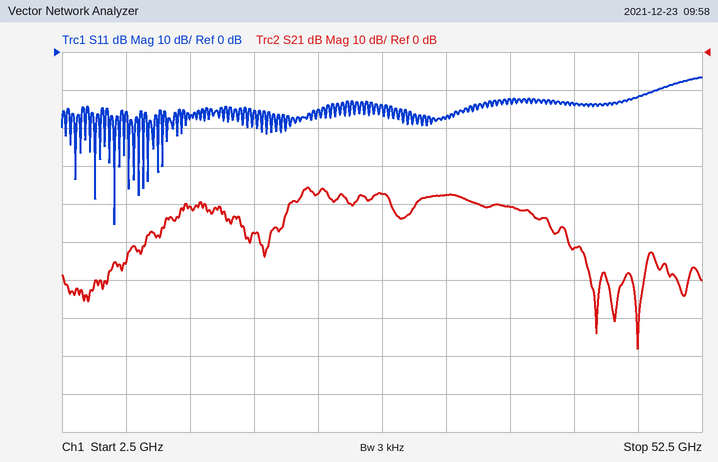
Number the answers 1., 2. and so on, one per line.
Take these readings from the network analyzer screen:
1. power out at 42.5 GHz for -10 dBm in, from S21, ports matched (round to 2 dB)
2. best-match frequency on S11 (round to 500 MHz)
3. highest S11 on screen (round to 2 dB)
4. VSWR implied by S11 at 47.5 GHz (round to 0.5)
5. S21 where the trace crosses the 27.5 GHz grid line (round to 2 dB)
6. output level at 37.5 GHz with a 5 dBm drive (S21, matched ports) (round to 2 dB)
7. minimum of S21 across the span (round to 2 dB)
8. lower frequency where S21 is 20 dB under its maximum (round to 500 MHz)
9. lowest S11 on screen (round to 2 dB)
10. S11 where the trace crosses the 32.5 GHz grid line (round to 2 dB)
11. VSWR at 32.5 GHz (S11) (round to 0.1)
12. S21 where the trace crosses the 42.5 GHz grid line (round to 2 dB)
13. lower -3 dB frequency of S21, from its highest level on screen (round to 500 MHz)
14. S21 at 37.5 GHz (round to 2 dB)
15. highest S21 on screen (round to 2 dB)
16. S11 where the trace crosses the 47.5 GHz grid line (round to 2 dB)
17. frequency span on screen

1. -62 dBm
2. 6.5 GHz
3. -6 dB
4. 1.5
5. -38 dB
6. -36 dBm
7. -78 dB
8. 7.5 GHz
9. -46 dB
10. -18 dB
11. 1.3
12. -52 dB
13. 21.0 GHz
14. -40 dB
15. -36 dB
16. -12 dB
17. 50 GHz
